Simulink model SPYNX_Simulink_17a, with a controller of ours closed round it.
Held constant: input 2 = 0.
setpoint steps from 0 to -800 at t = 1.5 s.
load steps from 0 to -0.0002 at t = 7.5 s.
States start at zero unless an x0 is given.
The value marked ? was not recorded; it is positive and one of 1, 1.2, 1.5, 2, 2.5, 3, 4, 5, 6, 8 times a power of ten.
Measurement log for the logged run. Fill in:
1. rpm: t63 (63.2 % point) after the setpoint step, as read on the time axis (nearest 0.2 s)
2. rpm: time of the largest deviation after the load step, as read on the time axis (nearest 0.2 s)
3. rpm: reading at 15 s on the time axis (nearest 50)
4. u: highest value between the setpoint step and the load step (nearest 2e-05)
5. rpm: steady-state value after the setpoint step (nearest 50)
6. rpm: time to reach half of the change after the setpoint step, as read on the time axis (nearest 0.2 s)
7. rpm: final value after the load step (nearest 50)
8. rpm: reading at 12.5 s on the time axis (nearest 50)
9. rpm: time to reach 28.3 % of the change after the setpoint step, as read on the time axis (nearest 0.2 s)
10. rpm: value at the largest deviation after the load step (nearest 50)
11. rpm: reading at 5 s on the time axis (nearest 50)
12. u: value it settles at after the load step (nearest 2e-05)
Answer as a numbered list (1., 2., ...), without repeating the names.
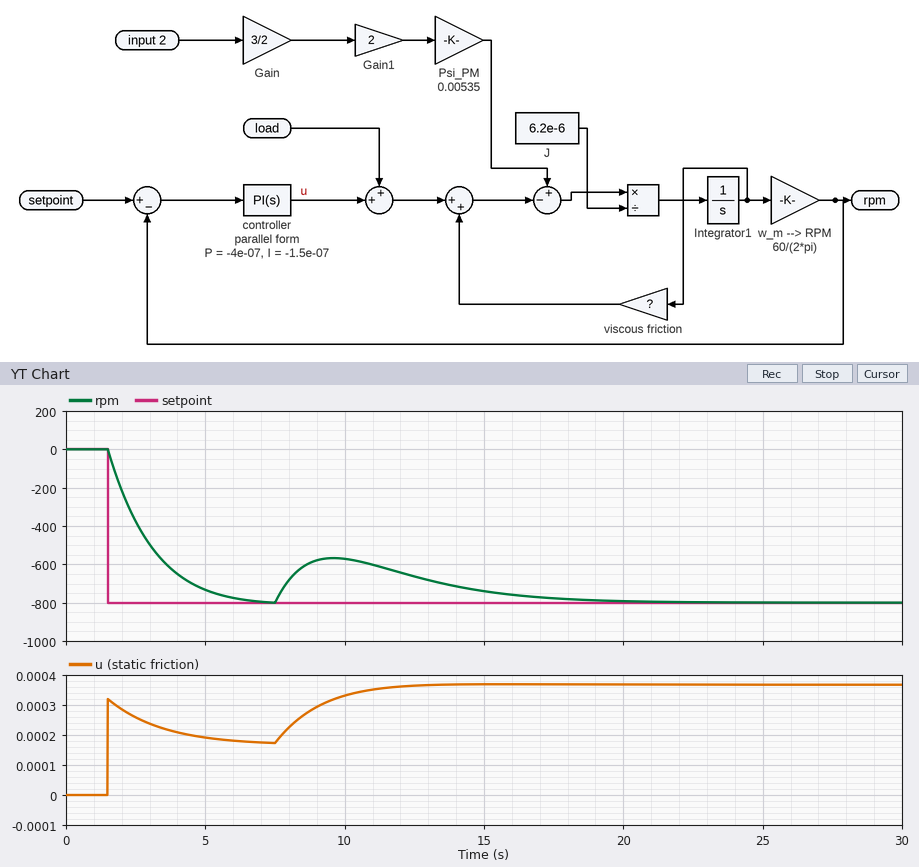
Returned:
1. 3.0 s
2. 9.6 s
3. -750
4. 0.00032
5. -800
6. 2.6 s
7. -800
8. -650
9. 2.0 s
10. -550
11. -750
12. 0.00036
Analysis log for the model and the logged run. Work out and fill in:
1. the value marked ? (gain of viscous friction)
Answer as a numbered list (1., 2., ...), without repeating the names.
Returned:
1. 2e-06
